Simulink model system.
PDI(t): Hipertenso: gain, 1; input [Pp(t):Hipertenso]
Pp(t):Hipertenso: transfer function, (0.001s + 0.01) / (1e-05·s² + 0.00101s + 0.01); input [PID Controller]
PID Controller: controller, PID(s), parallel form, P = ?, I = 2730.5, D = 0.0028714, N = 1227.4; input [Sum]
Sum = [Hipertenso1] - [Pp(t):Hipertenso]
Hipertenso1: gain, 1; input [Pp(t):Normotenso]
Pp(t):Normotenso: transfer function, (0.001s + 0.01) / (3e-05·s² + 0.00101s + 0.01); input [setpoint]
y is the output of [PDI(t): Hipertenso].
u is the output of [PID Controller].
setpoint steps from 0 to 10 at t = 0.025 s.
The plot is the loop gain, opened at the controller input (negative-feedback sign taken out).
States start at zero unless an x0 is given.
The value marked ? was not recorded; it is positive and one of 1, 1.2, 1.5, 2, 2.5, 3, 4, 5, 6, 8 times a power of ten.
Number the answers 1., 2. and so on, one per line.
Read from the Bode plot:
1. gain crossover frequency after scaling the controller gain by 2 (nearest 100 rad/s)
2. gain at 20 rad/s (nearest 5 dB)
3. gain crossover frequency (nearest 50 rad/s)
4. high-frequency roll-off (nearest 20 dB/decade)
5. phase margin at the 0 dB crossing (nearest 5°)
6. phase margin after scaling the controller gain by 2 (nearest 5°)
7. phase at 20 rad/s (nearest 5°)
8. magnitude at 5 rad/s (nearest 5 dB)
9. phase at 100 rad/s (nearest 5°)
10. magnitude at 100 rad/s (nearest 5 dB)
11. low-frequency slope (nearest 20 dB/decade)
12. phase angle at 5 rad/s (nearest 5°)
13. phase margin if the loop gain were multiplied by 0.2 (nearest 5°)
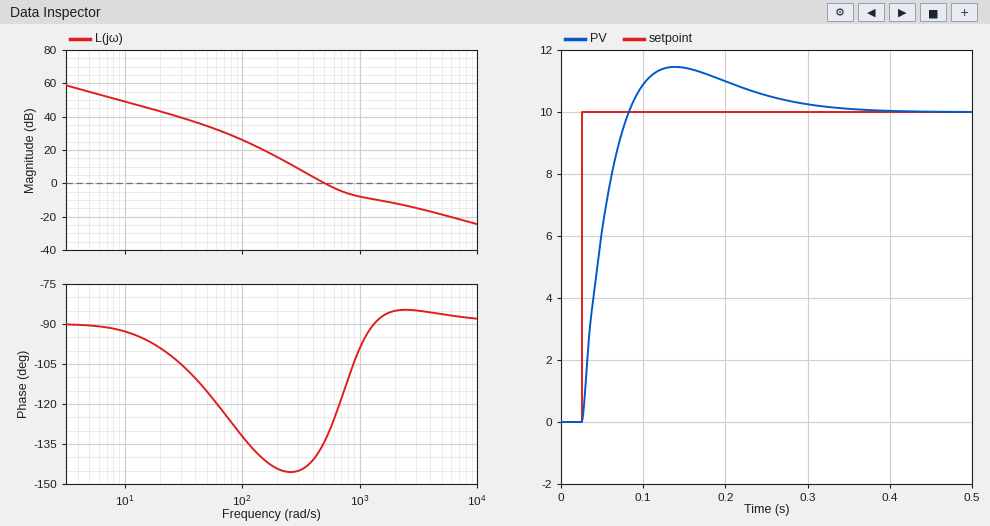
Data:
1. 800 rad/s
2. 45 dB
3. 500 rad/s
4. -20 dB/decade
5. 45°
6. 70°
7. -100°
8. 55 dB
9. -130°
10. 25 dB
11. -20 dB/decade
12. -90°
13. 35°
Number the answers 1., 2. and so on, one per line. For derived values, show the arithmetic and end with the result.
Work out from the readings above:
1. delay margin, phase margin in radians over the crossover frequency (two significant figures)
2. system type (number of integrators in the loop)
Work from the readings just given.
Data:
1. 45 × π / 180 / 500 = 0.0016 s
2. 1
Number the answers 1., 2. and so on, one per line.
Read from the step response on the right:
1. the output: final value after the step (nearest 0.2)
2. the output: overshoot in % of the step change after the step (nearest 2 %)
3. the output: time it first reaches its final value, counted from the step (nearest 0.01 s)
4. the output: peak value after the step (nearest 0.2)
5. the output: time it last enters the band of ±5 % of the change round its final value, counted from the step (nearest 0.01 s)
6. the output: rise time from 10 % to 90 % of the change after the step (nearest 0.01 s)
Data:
1. 10.0
2. 14 %
3. 0.06 s
4. 11.4
5. 0.23 s
6. 0.04 s
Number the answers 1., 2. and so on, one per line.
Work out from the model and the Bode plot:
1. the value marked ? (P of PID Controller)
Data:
1. 2.5
